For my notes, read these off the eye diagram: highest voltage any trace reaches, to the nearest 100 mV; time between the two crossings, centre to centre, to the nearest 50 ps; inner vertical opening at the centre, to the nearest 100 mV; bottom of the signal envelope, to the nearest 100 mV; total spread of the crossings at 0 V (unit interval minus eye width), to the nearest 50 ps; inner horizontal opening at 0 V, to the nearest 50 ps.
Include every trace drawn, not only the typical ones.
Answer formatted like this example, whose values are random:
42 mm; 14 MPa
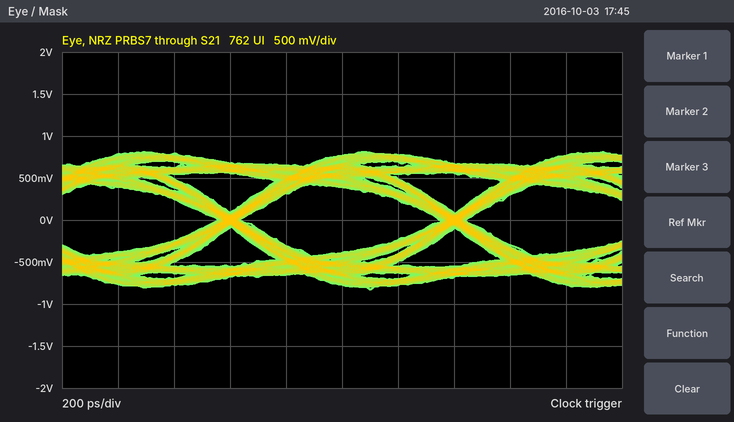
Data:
800 mV; 800 ps; 800 mV; -800 mV; 100 ps; 700 ps
